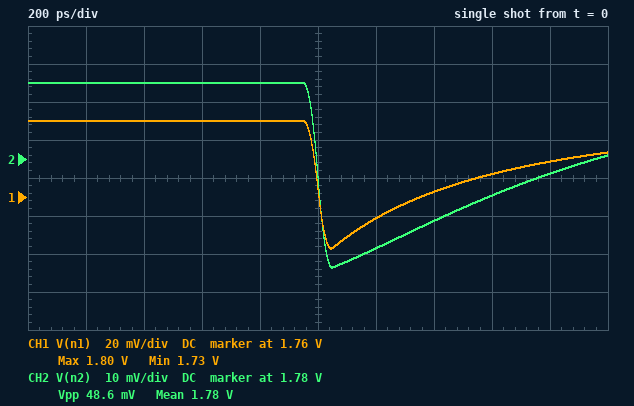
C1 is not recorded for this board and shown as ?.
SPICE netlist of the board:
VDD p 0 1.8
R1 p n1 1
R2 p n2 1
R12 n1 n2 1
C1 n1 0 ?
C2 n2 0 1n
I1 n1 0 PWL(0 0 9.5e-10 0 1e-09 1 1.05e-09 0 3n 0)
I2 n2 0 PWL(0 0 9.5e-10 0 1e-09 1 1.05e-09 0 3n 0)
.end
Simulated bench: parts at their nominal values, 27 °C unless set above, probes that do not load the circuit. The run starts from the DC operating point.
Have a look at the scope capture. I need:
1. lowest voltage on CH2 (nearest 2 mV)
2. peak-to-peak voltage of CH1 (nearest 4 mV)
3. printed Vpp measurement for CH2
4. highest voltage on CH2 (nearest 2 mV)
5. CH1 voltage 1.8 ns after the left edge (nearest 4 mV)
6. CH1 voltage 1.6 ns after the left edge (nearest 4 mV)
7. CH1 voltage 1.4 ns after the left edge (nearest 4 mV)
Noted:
1.752 V
68 mV
48.6 mV
1.800 V
1.780 V
1.772 V
1.764 V
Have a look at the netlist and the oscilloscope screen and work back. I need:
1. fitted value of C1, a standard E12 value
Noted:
680 pF
